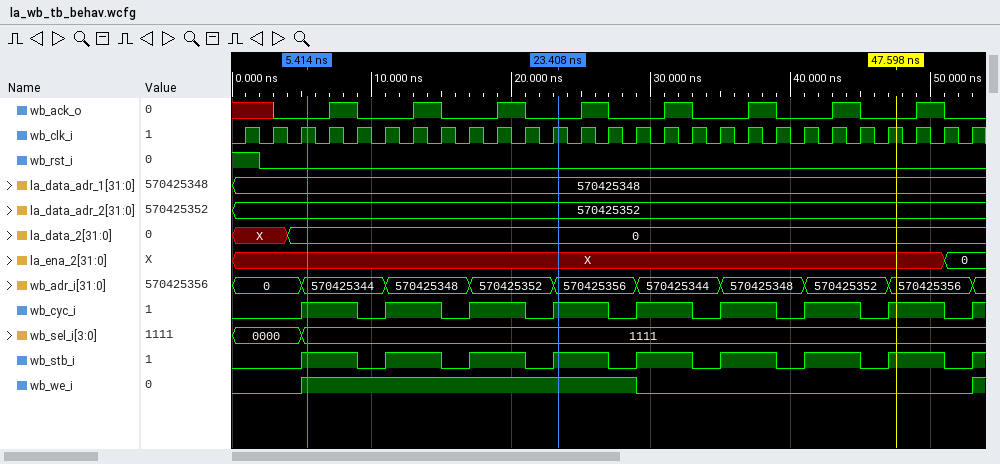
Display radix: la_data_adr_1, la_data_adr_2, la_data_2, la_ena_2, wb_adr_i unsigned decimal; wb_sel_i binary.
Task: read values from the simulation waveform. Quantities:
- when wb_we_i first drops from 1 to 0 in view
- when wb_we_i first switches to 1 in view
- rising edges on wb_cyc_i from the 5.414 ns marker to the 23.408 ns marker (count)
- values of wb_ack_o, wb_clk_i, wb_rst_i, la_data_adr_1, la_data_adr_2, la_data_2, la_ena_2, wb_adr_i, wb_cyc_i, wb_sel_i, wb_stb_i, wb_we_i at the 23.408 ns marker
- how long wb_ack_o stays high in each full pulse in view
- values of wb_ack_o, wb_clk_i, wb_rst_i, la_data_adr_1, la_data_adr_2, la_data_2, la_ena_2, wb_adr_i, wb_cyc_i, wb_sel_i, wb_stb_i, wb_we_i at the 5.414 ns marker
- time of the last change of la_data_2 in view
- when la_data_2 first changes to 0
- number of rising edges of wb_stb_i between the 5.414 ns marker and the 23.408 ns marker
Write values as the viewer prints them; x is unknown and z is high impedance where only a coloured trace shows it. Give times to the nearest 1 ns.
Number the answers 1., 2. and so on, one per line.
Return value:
1. 29 ns
2. 5 ns
3. 3
4. wb_ack_o=0, wb_clk_i=1, wb_rst_i=0, la_data_adr_1=570425348, la_data_adr_2=570425352, la_data_2=0, la_ena_2=X, wb_adr_i=570425356, wb_cyc_i=1, wb_sel_i=1111, wb_stb_i=1, wb_we_i=1
5. 2 ns, 2 ns, 2 ns, 2 ns, 2 ns, 2 ns, 2 ns, 2 ns
6. wb_ack_o=0, wb_clk_i=1, wb_rst_i=0, la_data_adr_1=570425348, la_data_adr_2=570425352, la_data_2=0, la_ena_2=X, wb_adr_i=570425344, wb_cyc_i=1, wb_sel_i=1111, wb_stb_i=1, wb_we_i=1
7. 4 ns
8. 4 ns
9. 3
